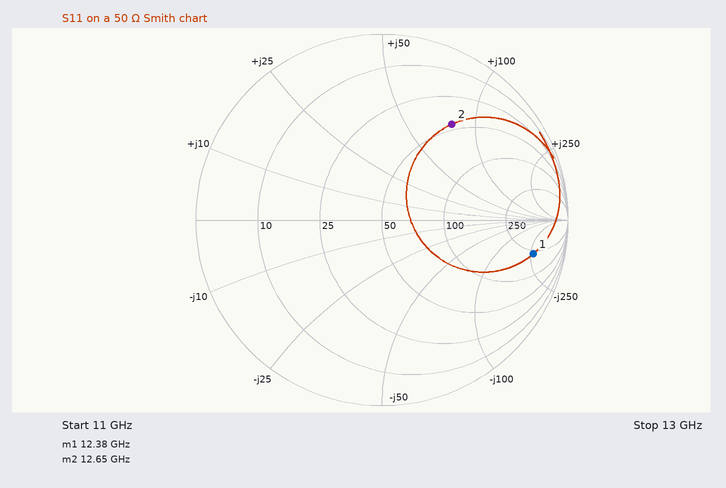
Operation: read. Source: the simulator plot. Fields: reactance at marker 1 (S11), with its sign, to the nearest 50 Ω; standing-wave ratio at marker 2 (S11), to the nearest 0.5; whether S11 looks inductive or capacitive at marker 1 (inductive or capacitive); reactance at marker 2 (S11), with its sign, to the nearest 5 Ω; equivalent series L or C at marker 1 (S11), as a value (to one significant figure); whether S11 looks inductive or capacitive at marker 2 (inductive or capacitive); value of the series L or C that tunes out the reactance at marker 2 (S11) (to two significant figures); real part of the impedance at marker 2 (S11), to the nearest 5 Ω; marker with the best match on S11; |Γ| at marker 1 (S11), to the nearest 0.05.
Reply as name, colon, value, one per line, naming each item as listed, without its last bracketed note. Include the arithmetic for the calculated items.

reactance at marker 1 (S11), with its sign, to the nearest 50 Ω: -250 Ω
standing-wave ratio at marker 2 (S11), to the nearest 0.5: 4.5
whether S11 looks inductive or capacitive at marker 1: capacitive
reactance at marker 2 (S11), with its sign, to the nearest 5 Ω: +80 Ω
equivalent series L or C at marker 1 (S11), as a value: C = 1/(2π × 12.38 GHz × 250 Ω) ≈ 51.4 fF, so 50 fF to one significant figure
whether S11 looks inductive or capacitive at marker 2: inductive
value of the series L or C that tunes out the reactance at marker 2 (S11): C = 1/(2π × 12.65 GHz × 80 Ω) ≈ 157 fF, so 160 fF to two significant figures
real part of the impedance at marker 2 (S11), to the nearest 5 Ω: 45 Ω
marker with the best match on S11: marker 2
|Γ| at marker 1 (S11), to the nearest 0.05: 0.85
